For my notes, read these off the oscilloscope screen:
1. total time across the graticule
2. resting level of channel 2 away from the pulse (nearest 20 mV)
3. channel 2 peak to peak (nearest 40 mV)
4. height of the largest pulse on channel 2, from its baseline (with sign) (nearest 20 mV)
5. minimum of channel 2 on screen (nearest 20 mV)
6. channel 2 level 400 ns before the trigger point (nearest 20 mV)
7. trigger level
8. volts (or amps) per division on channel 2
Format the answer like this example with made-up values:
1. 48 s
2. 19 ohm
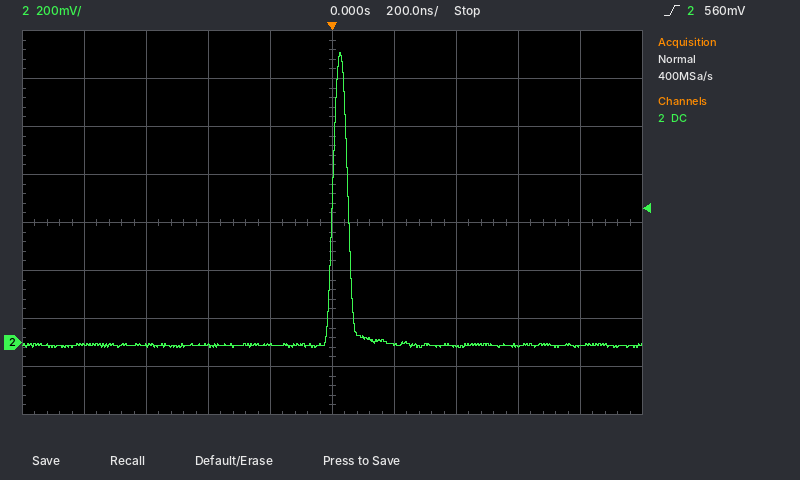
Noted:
1. 2 µs
2. -20 mV
3. 1.24 V
4. +1.22 V
5. -20 mV
6. -20 mV
7. 560 mV
8. 200 mV
